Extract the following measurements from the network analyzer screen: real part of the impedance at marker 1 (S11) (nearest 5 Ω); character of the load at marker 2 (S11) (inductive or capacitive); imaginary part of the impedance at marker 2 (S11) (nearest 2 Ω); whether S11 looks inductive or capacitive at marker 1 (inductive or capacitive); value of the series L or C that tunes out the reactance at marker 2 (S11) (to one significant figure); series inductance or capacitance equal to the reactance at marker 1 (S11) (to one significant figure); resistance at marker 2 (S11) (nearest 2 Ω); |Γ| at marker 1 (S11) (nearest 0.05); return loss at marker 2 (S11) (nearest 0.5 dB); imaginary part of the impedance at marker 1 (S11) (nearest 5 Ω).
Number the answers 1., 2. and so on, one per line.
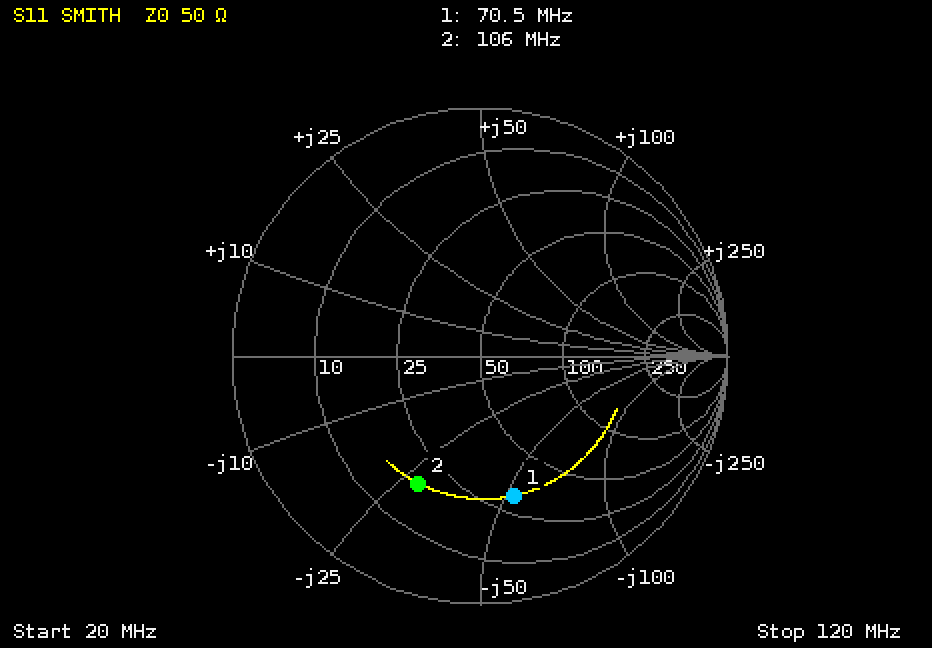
1. 30 Ω
2. capacitive
3. -28 Ω
4. capacitive
5. 40 nH
6. 40 pF
7. 18 Ω
8. 0.60
9. 5.0 dB
10. -55 Ω
